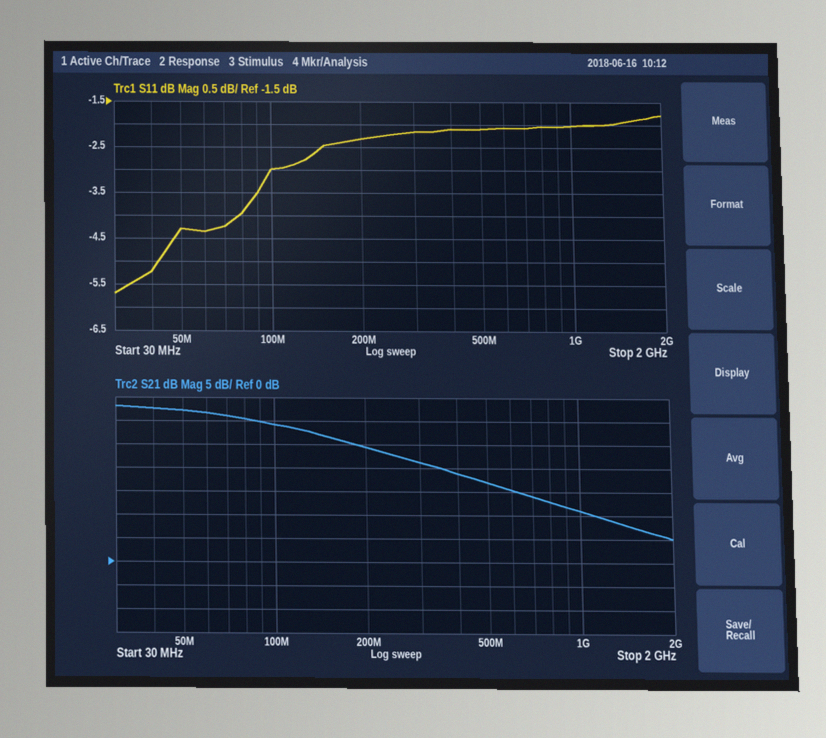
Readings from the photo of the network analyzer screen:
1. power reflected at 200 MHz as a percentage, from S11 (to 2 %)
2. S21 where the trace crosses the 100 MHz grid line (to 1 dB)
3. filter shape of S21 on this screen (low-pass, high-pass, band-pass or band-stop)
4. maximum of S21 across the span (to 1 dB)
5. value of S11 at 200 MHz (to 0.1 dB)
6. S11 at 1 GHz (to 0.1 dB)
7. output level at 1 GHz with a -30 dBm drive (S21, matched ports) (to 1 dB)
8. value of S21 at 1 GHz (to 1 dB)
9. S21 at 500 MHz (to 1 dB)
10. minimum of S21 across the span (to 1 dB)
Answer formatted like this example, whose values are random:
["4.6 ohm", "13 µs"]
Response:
["58 %", "29 dB", "low-pass", "33 dB", "-2.3 dB", "-2.0 dB", "-19 dBm", "11 dB", "17 dB", "5 dB"]
